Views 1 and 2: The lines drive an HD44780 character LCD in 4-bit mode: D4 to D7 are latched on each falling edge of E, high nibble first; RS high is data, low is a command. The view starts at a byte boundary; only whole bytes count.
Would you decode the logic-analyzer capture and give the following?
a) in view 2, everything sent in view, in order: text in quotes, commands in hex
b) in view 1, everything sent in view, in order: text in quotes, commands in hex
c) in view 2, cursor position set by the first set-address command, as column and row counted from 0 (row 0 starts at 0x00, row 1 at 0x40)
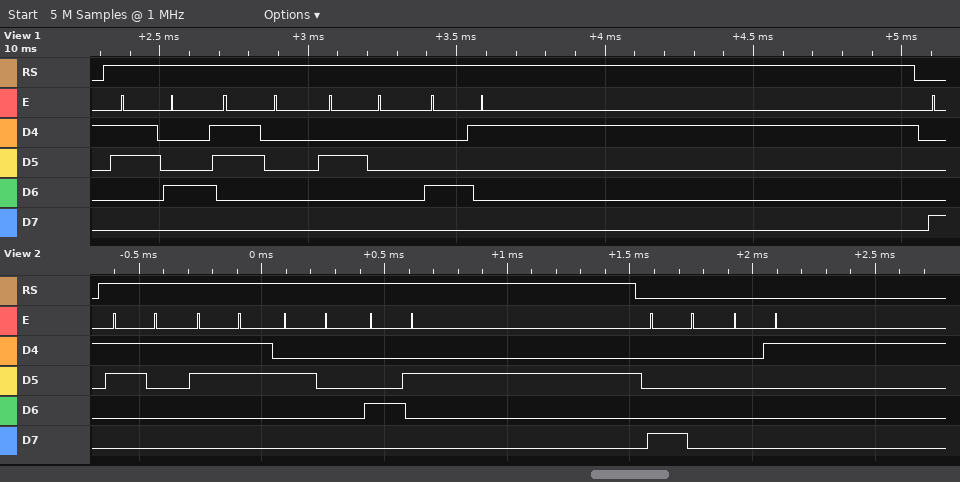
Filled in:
"13 B" 0x80 0x01
"40 A"
column 0, row 0
